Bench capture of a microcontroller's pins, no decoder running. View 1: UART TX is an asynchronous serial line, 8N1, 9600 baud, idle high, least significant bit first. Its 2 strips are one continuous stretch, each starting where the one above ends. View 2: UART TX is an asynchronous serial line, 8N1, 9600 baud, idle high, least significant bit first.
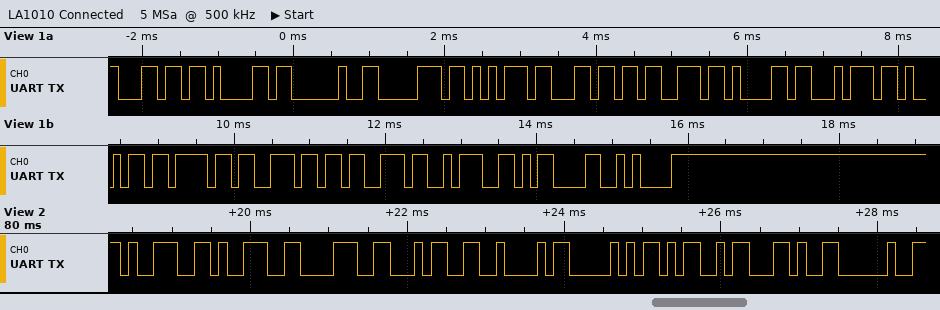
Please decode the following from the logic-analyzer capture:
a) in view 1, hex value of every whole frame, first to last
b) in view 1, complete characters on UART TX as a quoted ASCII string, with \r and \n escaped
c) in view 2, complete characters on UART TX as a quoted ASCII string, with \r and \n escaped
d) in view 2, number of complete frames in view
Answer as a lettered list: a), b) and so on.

a) 6C 61 20 70 75 6C 73 61 74 69 6F 6E 73 3A 0D 0A
b) "la pulsations:\r\n"
c) "9984BPM, "
d) 9
